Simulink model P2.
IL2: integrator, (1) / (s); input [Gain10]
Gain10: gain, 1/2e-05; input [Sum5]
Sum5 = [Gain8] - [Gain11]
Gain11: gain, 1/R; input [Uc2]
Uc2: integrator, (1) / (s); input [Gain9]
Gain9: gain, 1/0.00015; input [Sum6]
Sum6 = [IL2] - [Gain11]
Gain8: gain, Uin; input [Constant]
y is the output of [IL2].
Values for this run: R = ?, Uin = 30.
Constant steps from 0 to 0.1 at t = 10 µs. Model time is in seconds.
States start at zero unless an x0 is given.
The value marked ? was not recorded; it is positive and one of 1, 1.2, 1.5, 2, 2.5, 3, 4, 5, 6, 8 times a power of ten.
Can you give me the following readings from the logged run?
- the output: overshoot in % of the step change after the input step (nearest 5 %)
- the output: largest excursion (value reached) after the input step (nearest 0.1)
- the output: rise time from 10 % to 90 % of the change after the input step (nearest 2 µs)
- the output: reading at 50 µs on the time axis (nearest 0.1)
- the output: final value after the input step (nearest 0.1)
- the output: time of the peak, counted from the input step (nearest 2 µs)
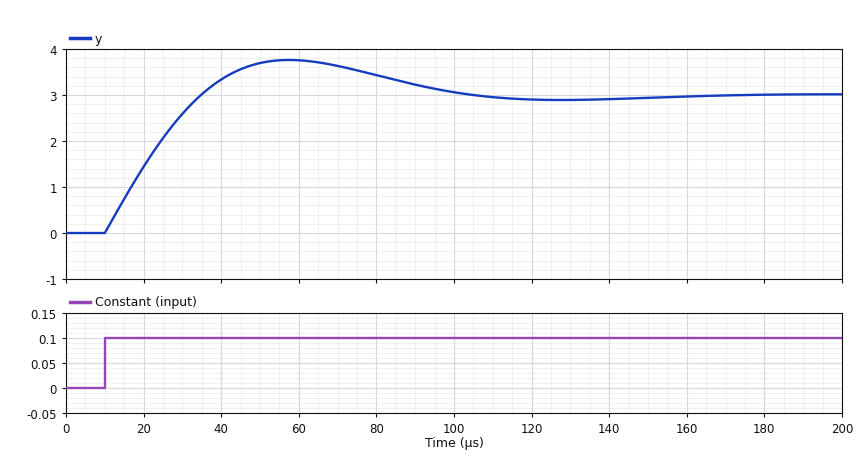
25 %
3.8
20 µs
3.7
3.0
48 µs
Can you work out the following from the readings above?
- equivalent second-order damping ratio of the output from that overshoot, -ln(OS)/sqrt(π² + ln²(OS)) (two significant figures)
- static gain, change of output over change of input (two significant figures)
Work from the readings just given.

0.40
30
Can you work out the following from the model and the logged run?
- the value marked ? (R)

0.12
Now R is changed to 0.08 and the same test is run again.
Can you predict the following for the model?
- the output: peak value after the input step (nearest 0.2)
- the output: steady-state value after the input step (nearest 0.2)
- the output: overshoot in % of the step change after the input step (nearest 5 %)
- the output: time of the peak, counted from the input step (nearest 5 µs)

3.4
3.0
10 %
45 µs
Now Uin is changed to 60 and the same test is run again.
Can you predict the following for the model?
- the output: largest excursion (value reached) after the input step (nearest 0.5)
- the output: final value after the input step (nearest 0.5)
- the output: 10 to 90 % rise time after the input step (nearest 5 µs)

7.5
6.0
20 µs
